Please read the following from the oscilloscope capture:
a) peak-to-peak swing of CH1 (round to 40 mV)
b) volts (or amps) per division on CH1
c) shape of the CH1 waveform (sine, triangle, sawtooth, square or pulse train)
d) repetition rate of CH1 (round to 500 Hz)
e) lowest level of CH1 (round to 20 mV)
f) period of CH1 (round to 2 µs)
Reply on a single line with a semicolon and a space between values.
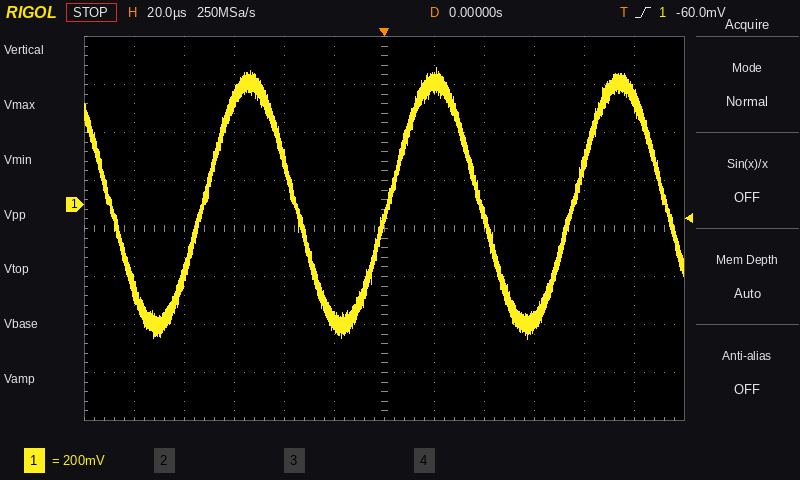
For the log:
1.12 V; 200 mV; sine; 13.5 kHz; -560 mV; 74 µs
